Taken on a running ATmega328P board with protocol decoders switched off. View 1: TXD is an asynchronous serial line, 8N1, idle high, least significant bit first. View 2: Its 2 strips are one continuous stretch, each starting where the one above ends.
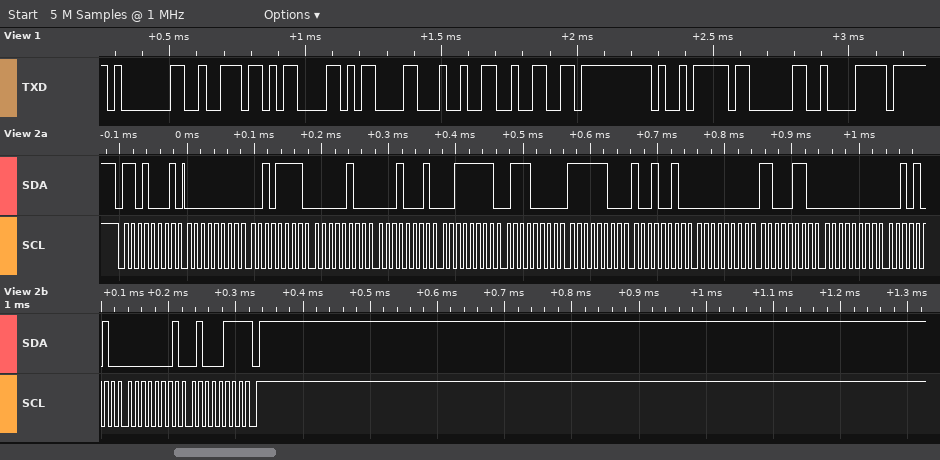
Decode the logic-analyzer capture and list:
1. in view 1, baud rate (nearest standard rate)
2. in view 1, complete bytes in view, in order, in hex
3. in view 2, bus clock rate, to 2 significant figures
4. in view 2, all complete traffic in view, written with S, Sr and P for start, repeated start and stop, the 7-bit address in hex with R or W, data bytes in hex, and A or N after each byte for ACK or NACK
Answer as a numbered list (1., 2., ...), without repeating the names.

1. 38400 baud
2. 01 72 0D 0D 24 32 FF E9 03 C2
3. 100 kHz
4. S 68R A 00 A 2F A 04 A 11 A 3F A 70 A FC A 92 A 00 A C6 A 00 A 2A A 01 A 47 N P
